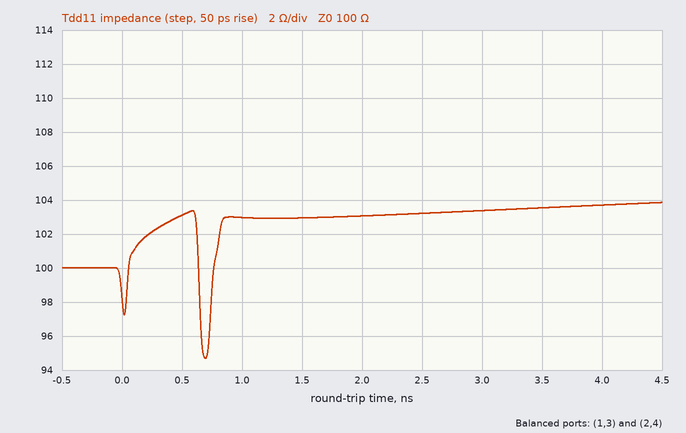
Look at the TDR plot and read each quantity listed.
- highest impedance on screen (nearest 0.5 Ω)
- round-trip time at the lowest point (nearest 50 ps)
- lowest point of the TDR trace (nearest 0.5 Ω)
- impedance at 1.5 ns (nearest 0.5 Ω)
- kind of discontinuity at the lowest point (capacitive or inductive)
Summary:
104.0 Ω
700 ps
94.5 Ω
103.0 Ω
capacitive
